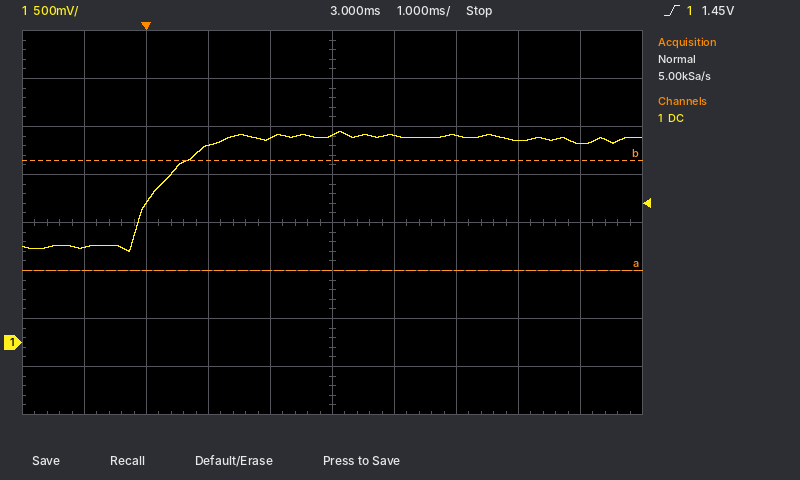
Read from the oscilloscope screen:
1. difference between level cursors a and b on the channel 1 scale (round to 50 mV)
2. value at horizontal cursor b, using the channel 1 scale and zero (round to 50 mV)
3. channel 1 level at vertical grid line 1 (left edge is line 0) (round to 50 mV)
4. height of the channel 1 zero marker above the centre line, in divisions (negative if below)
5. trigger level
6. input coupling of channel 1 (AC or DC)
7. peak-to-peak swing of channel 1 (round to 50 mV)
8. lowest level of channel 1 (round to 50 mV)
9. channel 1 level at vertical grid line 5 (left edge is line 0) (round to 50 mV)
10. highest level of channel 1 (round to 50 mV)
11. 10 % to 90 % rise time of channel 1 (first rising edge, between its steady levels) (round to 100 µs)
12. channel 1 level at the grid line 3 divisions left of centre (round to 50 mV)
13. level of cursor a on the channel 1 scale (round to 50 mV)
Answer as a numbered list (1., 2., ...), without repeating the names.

1. 1.15 V
2. 1.90 V
3. 1.00 V
4. -2.5 div
5. 1.45 V
6. DC
7. 1.25 V
8. 950 mV
9. 2.15 V
10. 2.20 V
11. 1.1 ms
12. 1.45 V
13. 750 mV
